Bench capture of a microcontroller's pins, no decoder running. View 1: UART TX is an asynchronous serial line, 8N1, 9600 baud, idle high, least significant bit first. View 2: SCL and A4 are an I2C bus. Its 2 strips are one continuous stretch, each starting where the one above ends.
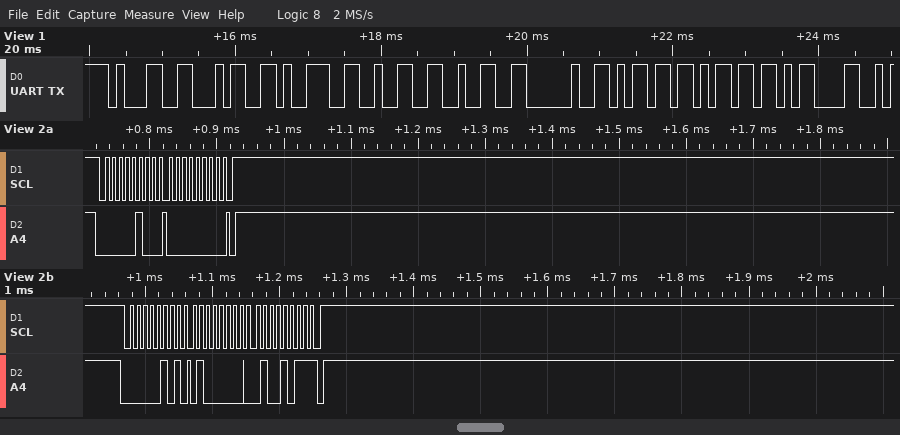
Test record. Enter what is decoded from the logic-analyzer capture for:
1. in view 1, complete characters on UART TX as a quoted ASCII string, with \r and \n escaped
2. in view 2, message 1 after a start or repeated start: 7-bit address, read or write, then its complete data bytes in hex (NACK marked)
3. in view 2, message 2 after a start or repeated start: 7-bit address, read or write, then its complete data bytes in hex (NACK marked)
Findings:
"14922 mm\r"
0x02 write: 00
0x02 read: 40 4B NACK
